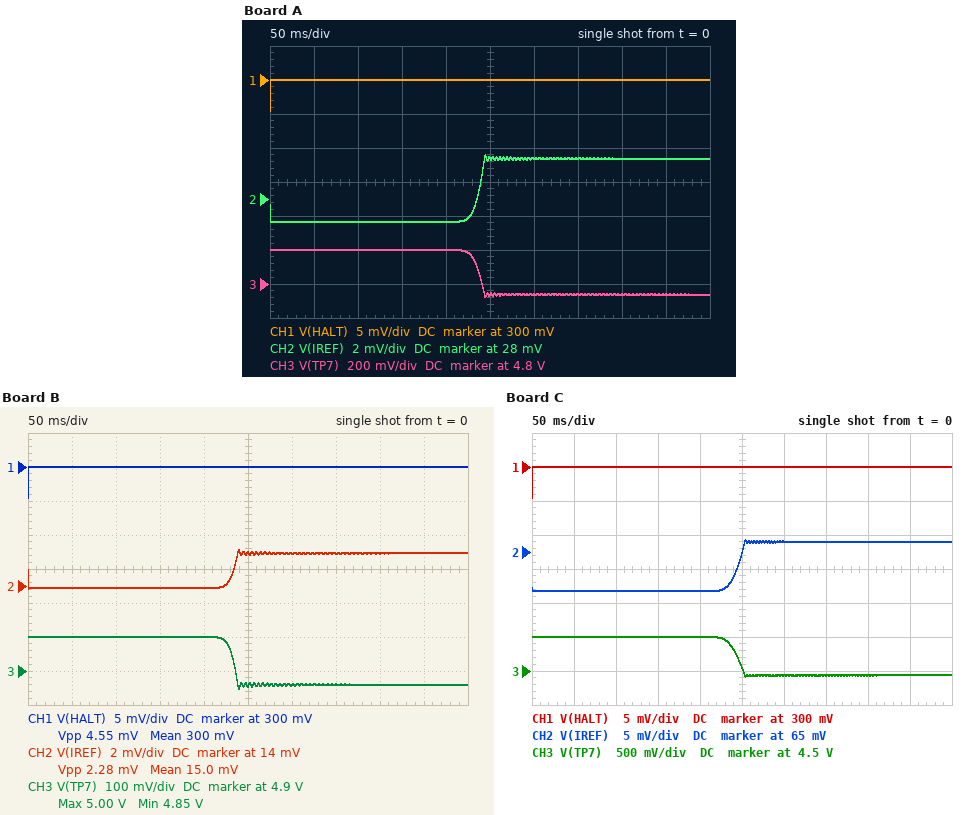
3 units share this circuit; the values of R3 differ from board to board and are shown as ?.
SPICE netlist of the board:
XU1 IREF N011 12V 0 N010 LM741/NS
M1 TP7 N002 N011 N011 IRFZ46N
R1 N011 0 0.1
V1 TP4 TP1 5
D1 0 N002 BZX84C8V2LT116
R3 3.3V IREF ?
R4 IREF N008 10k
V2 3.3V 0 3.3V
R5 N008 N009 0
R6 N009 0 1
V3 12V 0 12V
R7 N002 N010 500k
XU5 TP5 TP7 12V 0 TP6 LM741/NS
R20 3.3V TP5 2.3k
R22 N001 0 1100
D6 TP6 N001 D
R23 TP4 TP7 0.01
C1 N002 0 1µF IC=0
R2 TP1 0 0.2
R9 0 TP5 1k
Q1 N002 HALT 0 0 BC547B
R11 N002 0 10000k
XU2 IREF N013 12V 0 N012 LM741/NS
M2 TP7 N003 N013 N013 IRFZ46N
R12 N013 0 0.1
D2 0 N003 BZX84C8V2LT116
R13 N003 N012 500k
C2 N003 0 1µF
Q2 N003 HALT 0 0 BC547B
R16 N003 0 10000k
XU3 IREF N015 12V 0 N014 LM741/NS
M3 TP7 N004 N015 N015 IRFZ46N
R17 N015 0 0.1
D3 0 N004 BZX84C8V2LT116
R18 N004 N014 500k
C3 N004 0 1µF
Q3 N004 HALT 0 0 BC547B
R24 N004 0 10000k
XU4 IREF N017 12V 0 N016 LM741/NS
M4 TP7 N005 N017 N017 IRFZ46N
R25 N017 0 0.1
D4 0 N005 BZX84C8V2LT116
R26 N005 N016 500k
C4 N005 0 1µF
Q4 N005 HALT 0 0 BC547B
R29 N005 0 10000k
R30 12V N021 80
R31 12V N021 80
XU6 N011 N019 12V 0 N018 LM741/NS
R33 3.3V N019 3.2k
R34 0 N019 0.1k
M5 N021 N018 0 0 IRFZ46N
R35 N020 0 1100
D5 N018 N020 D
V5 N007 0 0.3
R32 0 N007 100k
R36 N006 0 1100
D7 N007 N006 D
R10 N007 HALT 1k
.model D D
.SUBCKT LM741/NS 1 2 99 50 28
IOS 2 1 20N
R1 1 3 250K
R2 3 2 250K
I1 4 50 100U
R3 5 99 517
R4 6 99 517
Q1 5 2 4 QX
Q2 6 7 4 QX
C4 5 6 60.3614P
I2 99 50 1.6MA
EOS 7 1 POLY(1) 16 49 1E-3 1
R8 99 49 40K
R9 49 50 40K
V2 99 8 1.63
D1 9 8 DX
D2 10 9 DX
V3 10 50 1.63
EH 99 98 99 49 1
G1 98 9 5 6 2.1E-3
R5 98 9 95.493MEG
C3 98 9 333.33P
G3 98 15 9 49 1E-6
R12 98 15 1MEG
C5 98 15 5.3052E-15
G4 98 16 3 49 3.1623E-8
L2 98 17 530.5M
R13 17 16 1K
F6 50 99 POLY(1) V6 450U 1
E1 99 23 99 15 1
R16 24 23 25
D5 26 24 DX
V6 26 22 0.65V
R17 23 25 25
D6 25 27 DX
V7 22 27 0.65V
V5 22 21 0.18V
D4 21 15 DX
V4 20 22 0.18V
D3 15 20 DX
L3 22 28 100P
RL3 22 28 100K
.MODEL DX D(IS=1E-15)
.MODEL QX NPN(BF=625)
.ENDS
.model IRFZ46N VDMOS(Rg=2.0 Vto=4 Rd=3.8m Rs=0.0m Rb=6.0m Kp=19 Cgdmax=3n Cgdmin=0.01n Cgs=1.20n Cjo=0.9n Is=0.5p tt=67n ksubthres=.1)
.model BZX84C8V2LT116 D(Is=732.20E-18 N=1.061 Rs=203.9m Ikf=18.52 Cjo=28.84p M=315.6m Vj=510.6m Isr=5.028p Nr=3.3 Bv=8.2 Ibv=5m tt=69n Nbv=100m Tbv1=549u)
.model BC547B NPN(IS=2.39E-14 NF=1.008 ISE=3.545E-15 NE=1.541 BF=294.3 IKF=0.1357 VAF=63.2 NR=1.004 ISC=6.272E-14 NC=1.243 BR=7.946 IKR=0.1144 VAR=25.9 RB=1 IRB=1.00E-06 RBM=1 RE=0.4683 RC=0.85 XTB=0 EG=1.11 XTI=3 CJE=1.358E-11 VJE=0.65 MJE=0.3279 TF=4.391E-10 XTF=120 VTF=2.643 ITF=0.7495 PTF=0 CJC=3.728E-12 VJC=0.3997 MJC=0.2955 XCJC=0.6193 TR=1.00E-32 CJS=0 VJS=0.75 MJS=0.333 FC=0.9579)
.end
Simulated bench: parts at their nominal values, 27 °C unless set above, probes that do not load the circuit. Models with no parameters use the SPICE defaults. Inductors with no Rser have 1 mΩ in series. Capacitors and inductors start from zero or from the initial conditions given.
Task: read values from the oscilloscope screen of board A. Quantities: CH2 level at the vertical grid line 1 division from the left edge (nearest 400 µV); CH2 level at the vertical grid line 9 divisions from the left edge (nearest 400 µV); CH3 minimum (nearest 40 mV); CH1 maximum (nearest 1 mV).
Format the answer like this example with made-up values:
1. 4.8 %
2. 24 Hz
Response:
1. 26.8 mV
2. 30.4 mV
3. 4.72 V
4. 300 mV
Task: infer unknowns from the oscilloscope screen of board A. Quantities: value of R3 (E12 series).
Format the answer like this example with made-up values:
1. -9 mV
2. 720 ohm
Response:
1. 1 MΩ
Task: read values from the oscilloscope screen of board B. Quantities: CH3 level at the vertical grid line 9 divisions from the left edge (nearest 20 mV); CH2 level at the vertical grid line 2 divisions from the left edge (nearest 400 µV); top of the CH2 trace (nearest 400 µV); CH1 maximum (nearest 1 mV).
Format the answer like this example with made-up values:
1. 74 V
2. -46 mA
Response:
1. 4.86 V
2. 14.0 mV
3. 16.0 mV
4. 300 mV
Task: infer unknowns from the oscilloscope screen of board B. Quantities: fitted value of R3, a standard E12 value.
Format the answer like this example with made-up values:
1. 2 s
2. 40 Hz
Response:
1. 1.8 MΩ
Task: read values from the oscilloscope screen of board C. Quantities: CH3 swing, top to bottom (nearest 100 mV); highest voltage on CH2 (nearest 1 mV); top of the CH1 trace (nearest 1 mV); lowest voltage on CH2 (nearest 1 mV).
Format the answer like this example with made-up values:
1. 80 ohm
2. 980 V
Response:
1. 600 mV
2. 67 mV
3. 300 mV
4. 59 mV
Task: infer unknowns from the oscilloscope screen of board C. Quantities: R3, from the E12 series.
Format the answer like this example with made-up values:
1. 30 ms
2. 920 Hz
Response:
1. 470 kΩ
